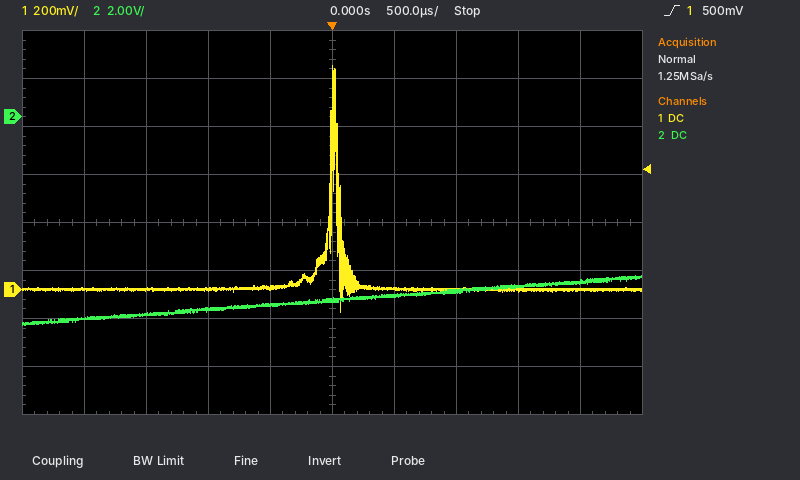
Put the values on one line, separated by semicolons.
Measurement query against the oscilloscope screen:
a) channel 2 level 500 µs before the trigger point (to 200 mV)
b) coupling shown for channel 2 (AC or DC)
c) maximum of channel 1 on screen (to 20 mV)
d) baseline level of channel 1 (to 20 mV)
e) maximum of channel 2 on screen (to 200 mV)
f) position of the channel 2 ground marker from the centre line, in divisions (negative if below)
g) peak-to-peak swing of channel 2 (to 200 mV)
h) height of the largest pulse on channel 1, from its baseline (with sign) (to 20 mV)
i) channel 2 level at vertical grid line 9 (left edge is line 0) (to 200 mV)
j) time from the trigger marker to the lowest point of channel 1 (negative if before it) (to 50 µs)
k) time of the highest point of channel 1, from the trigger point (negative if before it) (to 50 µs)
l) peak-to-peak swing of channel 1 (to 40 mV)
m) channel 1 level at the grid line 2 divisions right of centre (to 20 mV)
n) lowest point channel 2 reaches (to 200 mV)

-7.8 V; DC; 940 mV; 0 mV; -6.6 V; +2.2 div; 2.0 V; +940 mV; -6.8 V; +50 µs; 0 µs; 1.04 V; 0 mV; -8.6 V
